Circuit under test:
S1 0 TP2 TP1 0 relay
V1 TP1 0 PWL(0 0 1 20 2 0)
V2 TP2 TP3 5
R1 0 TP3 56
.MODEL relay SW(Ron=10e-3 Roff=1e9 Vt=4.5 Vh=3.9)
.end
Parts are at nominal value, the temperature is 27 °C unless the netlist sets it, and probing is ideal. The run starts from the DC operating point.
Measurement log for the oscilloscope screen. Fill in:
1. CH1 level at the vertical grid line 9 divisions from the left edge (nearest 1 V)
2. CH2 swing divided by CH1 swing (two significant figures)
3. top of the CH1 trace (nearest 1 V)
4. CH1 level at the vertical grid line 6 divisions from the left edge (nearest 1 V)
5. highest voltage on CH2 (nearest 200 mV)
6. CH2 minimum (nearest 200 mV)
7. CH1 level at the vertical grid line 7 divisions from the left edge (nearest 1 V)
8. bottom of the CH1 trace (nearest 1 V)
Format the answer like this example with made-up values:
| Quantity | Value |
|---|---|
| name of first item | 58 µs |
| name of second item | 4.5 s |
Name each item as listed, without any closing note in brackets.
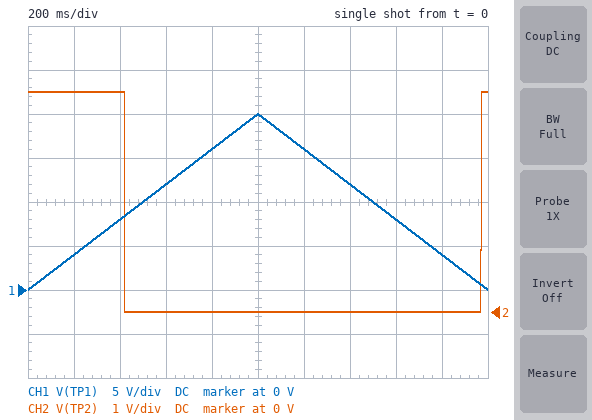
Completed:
| Quantity | Value |
|---|---|
| CH1 level at the vertical grid line 9 divisions from the left edge | 4 V |
| CH2 swing divided by CH1 swing | 0.25 |
| top of the CH1 trace | 20 V |
| CH1 level at the vertical grid line 6 divisions from the left edge | 16 V |
| highest voltage on CH2 | 5.0 V |
| CH2 minimum | 0 V |
| CH1 level at the vertical grid line 7 divisions from the left edge | 12 V |
| bottom of the CH1 trace | 0 V |
